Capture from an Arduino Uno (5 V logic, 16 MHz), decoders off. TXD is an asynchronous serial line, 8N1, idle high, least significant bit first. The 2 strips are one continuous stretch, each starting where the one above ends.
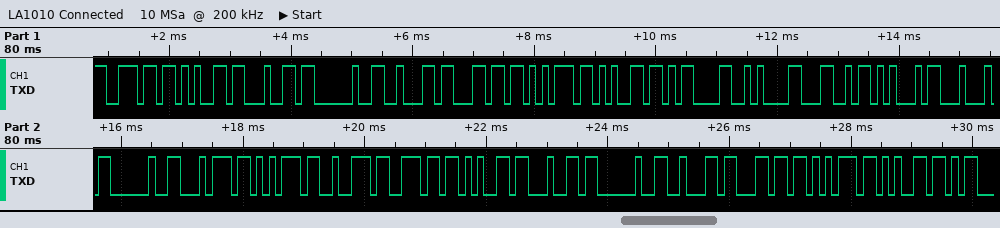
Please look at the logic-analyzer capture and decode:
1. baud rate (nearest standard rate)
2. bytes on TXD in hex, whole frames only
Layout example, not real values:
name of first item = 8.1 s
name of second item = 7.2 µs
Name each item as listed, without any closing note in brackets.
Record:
baud rate = 9600 baud
bytes on TXD in hex, whole frames only = 6E 65 64 20 62 6C 75 65 0D 0A 4C 45 44 20 74 75 72 6E 65 64 20 62 6C 75 65
